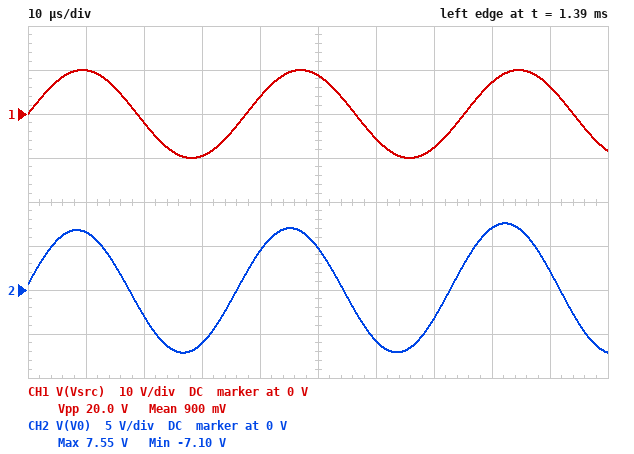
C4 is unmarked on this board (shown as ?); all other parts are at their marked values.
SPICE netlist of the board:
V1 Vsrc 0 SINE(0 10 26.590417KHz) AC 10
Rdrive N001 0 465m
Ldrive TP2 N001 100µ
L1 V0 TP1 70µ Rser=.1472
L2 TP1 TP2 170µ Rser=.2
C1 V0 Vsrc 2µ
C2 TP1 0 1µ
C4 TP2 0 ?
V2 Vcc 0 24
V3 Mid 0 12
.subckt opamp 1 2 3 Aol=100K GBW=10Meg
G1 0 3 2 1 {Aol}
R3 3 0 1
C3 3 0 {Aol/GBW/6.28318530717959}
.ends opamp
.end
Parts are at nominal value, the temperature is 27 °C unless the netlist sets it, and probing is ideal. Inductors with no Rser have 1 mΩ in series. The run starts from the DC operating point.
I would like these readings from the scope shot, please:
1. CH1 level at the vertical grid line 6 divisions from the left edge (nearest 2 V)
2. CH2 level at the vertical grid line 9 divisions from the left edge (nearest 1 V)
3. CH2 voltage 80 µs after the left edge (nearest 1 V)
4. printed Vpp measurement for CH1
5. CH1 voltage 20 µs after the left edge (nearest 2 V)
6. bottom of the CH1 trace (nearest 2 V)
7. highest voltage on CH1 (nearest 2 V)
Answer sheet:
-6 V
2 V
7 V
20.0 V
-2 V
-10 V
10 V
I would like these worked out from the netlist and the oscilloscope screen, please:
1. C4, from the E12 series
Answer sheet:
680 nF
